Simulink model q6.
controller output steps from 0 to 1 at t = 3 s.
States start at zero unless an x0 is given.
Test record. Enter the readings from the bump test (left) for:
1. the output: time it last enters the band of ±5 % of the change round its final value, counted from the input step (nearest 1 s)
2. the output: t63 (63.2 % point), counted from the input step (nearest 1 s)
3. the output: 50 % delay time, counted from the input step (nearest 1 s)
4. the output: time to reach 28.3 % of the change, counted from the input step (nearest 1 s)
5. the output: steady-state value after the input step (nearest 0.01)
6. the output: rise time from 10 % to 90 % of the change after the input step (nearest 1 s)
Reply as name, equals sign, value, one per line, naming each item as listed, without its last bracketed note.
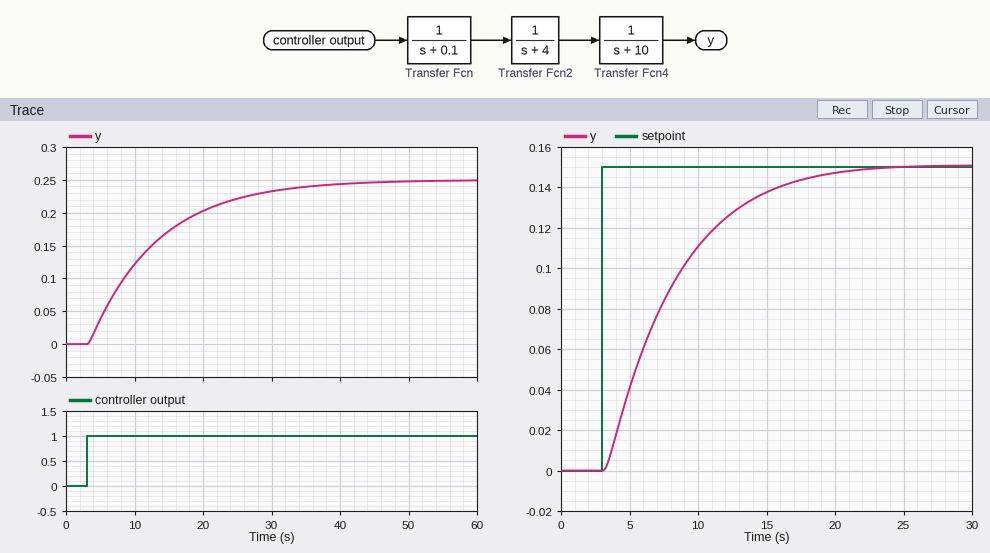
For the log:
the output: time it last enters the band of ±5 % of the change round its final value, counted from the input step = 30 s
the output: t63 (63.2 % point), counted from the input step = 10 s
the output: 50 % delay time, counted from the input step = 7 s
the output: time to reach 28.3 % of the change, counted from the input step = 4 s
the output: steady-state value after the input step = 0.25
the output: rise time from 10 % to 90 % of the change after the input step = 22 s
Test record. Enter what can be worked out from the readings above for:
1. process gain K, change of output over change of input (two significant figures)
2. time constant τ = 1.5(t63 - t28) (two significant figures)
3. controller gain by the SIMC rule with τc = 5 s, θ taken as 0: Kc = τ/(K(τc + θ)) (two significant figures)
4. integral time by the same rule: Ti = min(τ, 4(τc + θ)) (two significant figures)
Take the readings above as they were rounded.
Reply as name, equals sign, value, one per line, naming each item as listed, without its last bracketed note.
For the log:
process gain K, change of output over change of input = 0.25
time constant τ = 1.5(t63 - t28) = 9.0 s
controller gain by the SIMC rule with τc = 5 s, θ taken as 0: Kc = τ/(K(τc + θ)) = 7.2
integral time by the same rule: Ti = min(τ, 4(τc + θ)) = 9.0 s
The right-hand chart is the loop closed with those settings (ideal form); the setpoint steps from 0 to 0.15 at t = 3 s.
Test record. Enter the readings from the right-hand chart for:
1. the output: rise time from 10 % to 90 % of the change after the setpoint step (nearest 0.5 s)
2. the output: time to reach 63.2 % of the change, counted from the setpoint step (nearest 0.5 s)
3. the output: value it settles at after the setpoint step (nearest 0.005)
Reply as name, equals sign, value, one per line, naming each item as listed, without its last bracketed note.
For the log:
the output: rise time from 10 % to 90 % of the change after the setpoint step = 10.5 s
the output: time to reach 63.2 % of the change, counted from the setpoint step = 5.5 s
the output: value it settles at after the setpoint step = 0.150
